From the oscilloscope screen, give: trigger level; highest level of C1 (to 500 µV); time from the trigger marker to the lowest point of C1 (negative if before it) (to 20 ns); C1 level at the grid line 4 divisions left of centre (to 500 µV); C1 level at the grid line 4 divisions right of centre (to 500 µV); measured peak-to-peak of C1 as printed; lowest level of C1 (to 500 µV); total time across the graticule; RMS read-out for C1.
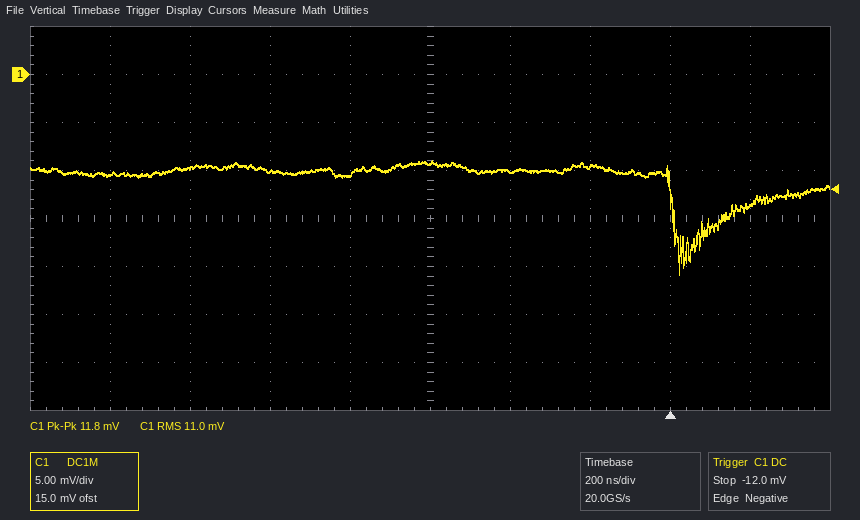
-12.0 mV
-9.0 mV
+20 ns
-10.5 mV
-13.5 mV
11.8 mV
-21.0 mV
2 µs
11.0 mV
